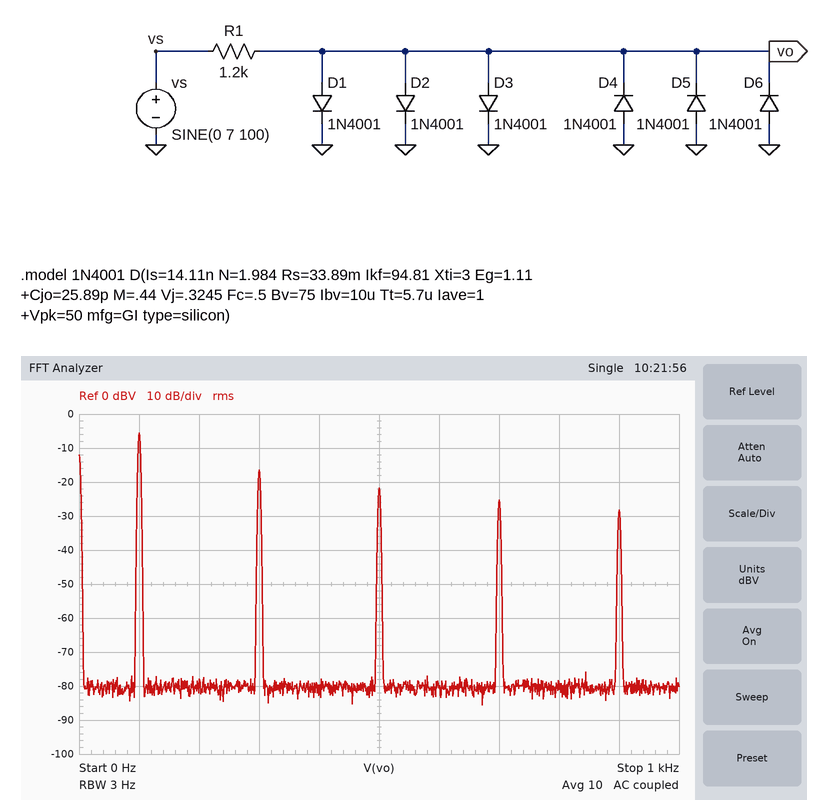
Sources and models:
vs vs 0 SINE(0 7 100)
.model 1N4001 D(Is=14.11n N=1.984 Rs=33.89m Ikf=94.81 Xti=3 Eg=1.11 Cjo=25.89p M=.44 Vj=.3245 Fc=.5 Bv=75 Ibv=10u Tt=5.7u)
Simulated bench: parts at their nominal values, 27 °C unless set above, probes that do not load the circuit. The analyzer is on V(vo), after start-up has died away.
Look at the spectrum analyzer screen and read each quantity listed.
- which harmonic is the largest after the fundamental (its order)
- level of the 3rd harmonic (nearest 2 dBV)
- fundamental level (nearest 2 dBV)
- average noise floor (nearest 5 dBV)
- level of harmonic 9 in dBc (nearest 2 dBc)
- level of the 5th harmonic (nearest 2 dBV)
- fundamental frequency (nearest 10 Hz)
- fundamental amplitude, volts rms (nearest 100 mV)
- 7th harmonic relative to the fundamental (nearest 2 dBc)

3
-16 dBV
-6 dBV
-80 dBV
-22 dBc
-22 dBV
100 Hz
500 mV
-20 dBc
